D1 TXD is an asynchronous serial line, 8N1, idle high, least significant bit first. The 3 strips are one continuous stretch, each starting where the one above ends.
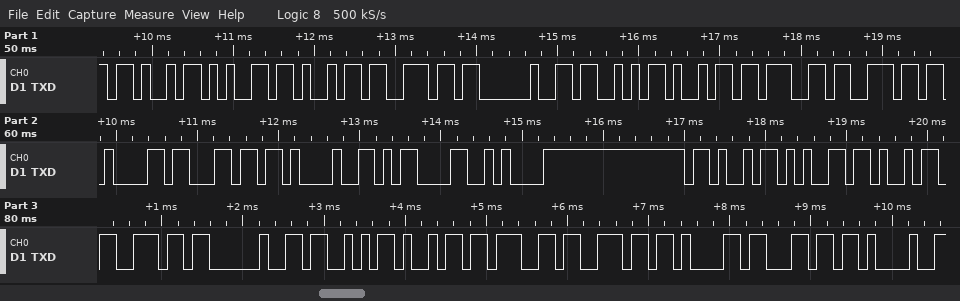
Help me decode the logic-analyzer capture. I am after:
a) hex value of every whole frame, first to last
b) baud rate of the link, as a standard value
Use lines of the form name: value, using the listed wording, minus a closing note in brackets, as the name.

hex value of every whole frame, first to last: 4B 65 69 6E 20 53 69 67 6E 61 6C 21 0D 0A 4B 65 69 6E 20 53 69 67 6E 61 6C 21
baud rate of the link, as a standard value: 9600 baud
